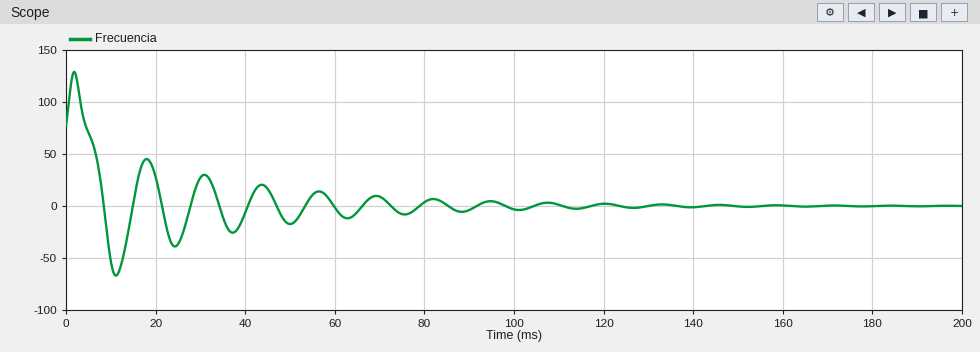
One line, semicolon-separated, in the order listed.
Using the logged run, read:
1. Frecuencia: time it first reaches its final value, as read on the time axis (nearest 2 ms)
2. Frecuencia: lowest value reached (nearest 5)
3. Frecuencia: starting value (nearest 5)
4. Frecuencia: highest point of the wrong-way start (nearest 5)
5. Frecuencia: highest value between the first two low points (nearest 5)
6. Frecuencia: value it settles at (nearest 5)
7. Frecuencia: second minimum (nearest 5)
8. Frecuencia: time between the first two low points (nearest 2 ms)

8 ms; -65; 75; 130; 45; 0; -40; 14 ms
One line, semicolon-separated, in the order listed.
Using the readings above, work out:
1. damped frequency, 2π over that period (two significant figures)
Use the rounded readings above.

0.45 rad/ms
